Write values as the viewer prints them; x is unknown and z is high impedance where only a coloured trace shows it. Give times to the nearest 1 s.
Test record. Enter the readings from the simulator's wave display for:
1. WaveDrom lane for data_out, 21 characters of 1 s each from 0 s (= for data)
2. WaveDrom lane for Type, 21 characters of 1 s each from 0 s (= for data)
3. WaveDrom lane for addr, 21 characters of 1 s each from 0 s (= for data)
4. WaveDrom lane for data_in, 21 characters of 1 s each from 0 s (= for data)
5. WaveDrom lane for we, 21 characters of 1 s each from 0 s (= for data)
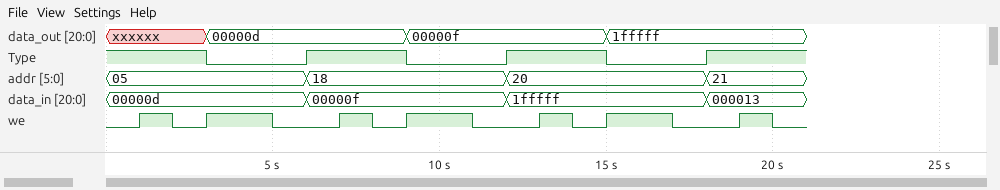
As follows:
{name: 'data_out', wave: 'x..=.....=.....=.....', data: '00000d 00000f 1fffff'}
{name: 'Type', wave: '1..0..1..0..1..0..1..'}
{name: 'addr', wave: '=.....=.....=.....=..', data: '05 18 20 21'}
{name: 'data_in', wave: '=.....=.....=.....=..', data: '00000d 00000f 1fffff 000013'}
{name: 'we', wave: '0101.0.101.0.101.0.10'}
